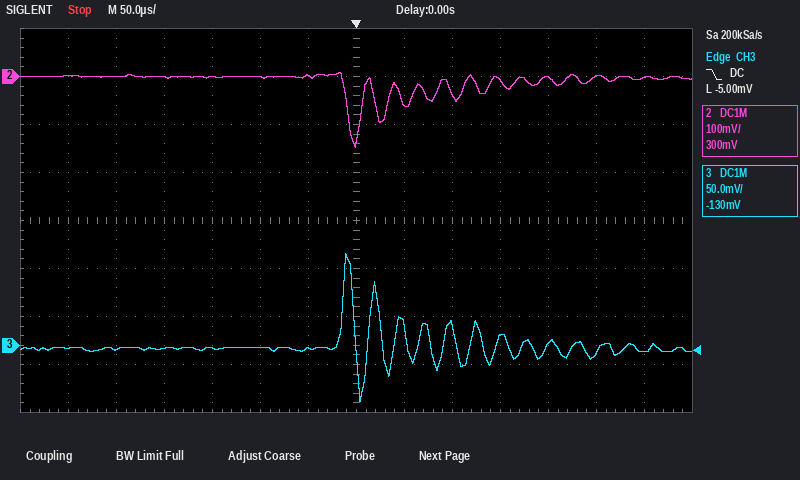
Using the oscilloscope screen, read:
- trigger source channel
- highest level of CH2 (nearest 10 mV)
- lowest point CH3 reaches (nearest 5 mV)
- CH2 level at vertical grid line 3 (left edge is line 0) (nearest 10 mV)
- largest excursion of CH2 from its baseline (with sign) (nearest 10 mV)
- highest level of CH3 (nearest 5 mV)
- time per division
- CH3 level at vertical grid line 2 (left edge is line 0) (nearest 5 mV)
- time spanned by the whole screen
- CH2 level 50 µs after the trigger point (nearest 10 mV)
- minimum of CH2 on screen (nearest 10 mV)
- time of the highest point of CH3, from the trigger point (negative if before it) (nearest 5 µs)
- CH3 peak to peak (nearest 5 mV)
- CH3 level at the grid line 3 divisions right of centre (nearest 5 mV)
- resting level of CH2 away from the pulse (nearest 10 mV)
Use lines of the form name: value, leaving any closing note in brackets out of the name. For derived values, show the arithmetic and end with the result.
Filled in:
trigger source channel: CH3
highest level of CH2: 10 mV
lowest point CH3 reaches: -60 mV
CH2 level at vertical grid line 3 (left edge is line 0): 0 mV
largest excursion of CH2 from its baseline (with sign): -150 mV − (0 mV) = -150 mV
highest level of CH3: 95 mV
time per division: 50 µs
CH3 level at vertical grid line 2 (left edge is line 0): -5 mV
time spanned by the whole screen: 700 µs
CH2 level 50 µs after the trigger point: -60 mV
minimum of CH2 on screen: -150 mV
time of the highest point of CH3, from the trigger point (negative if before it): -10 µs
CH3 peak to peak: 95 mV − (-60 mV) = 155 mV
CH3 level at the grid line 3 divisions right of centre: 10 mV
resting level of CH2 away from the pulse: 0 mV
